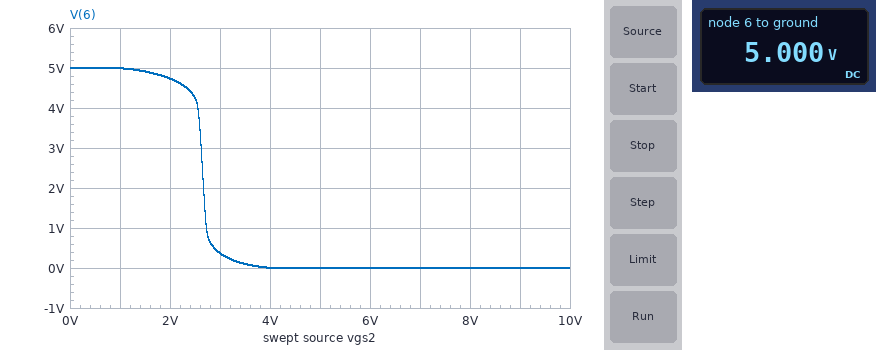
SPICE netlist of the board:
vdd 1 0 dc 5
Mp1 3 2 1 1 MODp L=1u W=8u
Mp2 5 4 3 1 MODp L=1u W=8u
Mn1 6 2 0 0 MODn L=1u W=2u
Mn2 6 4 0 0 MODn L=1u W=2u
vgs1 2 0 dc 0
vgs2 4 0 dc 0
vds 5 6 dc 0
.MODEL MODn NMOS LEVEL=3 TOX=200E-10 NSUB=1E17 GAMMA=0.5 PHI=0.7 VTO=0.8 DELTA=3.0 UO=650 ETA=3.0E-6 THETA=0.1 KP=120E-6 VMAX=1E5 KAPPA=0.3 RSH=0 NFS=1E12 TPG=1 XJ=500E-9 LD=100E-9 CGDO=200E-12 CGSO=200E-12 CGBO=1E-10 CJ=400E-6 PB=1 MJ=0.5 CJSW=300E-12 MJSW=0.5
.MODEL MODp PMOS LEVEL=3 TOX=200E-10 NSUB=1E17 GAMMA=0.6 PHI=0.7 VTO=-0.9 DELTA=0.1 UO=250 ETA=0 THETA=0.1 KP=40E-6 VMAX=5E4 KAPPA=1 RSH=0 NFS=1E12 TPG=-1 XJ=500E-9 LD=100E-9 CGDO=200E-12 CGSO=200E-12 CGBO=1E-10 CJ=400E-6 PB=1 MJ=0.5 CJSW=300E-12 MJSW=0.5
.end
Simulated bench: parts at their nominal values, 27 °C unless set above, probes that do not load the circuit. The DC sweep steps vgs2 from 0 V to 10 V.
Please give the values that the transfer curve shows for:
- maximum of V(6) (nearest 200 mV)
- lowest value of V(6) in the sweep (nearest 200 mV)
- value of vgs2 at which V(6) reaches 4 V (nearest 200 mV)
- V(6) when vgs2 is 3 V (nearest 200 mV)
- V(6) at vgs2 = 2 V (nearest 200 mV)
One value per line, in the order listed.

5.0 V
0 V
2.6 V
400 mV
4.8 V
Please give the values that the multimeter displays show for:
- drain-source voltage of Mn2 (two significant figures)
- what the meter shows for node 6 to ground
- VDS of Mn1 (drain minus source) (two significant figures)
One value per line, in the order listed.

5.0 V
5.000 V
5.0 V
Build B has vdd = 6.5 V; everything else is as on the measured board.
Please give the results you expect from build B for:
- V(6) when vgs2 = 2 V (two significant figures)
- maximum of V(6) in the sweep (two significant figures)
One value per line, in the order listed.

6.3 V
6.5 V
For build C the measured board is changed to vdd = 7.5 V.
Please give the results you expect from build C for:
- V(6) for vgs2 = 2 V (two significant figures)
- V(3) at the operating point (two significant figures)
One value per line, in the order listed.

7.3 V
7.5 V
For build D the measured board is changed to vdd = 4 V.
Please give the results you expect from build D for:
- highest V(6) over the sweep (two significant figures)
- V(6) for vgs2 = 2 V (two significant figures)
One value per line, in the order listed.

4.0 V
3.4 V
